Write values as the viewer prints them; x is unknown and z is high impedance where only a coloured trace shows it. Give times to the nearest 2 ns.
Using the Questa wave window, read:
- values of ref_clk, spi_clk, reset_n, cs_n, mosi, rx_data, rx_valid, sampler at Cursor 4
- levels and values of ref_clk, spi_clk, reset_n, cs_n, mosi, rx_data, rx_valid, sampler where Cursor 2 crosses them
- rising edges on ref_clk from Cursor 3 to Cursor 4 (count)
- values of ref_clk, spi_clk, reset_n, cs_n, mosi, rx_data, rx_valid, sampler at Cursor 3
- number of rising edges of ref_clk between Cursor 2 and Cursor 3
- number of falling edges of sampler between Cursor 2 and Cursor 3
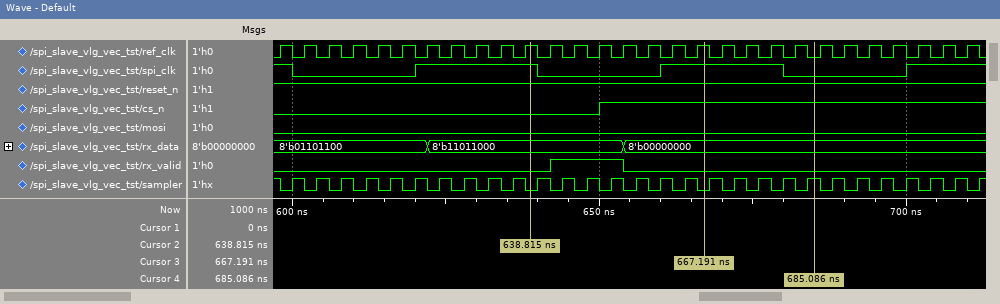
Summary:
ref_clk=0, spi_clk=0, reset_n=1, cs_n=1, mosi=0, rx_data=8'b00000000, rx_valid=0, sampler=1
ref_clk=1, spi_clk=1, reset_n=1, cs_n=0, mosi=0, rx_data=8'b11011000, rx_valid=0, sampler=0
4
ref_clk=1, spi_clk=1, reset_n=1, cs_n=1, mosi=0, rx_data=8'b00000000, rx_valid=0, sampler=0
7
7
